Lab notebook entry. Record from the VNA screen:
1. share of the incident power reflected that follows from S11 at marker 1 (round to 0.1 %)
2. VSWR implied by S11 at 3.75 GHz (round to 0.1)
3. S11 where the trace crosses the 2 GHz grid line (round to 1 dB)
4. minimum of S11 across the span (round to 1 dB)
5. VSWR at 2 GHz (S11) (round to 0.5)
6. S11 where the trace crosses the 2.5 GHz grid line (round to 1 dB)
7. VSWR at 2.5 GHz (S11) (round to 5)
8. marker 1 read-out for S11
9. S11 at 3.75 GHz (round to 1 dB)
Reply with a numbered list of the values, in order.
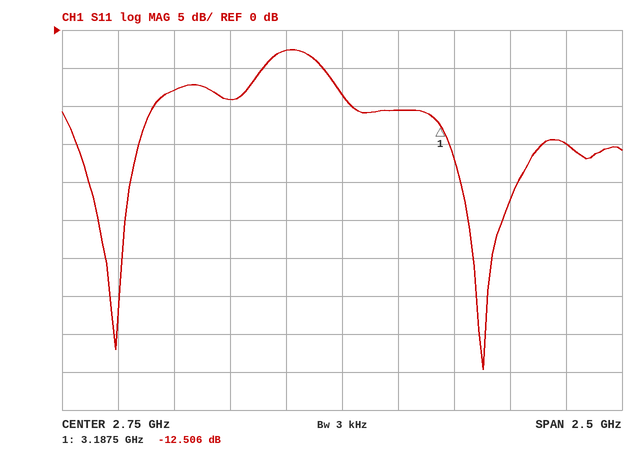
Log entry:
1. 5.6 %
2. 1.4
3. -8 dB
4. -45 dB
5. 2.5
6. -3 dB
7. 5
8. -12.506 dB
9. -15 dB
